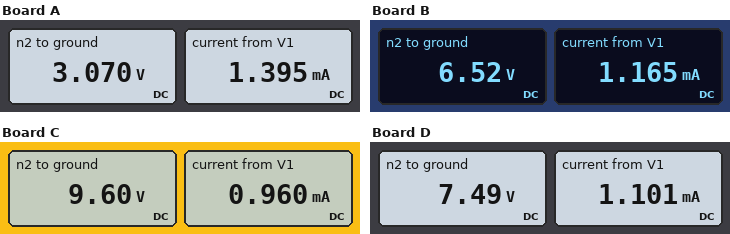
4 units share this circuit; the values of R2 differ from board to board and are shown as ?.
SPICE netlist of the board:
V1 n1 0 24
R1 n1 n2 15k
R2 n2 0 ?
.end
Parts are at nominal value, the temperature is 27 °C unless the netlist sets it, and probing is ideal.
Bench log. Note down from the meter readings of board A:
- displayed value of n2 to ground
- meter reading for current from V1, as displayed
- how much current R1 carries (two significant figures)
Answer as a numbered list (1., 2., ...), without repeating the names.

1. 3.070 V
2. 1.395 mA
3. 1.4 mA
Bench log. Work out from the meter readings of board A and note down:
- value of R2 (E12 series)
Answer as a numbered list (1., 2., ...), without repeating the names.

1. 2.2 kΩ
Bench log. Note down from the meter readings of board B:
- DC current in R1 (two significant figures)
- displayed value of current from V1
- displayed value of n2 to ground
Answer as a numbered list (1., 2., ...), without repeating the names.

1. 1.2 mA
2. 1.165 mA
3. 6.52 V
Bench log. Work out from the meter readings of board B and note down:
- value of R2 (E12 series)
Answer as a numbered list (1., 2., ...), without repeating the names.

1. 5.6 kΩ
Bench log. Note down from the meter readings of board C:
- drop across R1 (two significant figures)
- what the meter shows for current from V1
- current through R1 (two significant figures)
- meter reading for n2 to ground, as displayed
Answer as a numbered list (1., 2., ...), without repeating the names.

1. 14 V
2. 0.960 mA
3. 960 µA
4. 9.60 V
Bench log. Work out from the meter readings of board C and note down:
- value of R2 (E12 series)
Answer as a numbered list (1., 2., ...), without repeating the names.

1. 10 kΩ
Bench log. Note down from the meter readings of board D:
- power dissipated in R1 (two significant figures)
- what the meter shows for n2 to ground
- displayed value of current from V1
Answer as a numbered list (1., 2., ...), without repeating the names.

1. 18 mW
2. 7.49 V
3. 1.101 mA
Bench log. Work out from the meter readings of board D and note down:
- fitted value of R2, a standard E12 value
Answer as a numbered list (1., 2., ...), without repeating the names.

1. 6.8 kΩ
